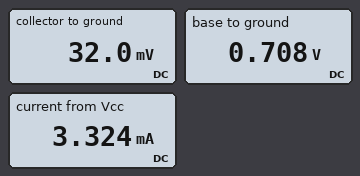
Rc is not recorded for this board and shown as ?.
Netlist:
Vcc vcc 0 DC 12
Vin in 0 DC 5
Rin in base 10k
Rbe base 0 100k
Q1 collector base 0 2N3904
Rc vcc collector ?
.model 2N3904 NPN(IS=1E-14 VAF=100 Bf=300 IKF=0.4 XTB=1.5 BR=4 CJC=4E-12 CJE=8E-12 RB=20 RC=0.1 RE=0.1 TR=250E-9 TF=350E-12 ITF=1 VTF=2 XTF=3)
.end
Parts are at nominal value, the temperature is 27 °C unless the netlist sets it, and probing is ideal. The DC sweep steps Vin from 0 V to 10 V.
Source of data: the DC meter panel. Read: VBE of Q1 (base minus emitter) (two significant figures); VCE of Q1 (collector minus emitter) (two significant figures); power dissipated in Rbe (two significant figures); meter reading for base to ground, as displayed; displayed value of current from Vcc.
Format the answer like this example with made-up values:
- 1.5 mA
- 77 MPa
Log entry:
- 710 mV
- 32 mV
- 5.0 µW
- 0.708 V
- 3.324 mA
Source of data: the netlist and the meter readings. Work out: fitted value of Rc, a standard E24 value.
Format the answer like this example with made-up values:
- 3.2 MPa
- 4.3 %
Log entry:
- 3.6 kΩ
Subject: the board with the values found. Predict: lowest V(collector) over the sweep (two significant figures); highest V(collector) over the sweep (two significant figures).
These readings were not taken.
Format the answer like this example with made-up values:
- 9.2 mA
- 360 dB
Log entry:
- 21 mV
- 12 V
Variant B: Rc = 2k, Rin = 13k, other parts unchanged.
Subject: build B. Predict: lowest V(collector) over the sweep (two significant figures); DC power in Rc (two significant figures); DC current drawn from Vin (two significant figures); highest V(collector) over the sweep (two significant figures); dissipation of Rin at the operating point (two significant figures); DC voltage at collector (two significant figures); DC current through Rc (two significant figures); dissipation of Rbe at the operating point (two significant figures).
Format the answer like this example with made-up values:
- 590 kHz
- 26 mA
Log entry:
- 34 mV
- 71 mW
- 330 µA
- 12 V
- 1.4 mW
- 49 mV
- 6.0 mA
- 5.1 µW
